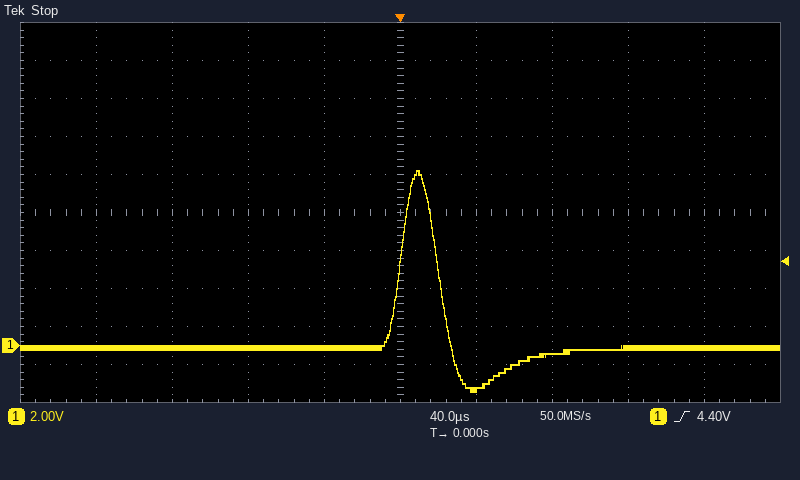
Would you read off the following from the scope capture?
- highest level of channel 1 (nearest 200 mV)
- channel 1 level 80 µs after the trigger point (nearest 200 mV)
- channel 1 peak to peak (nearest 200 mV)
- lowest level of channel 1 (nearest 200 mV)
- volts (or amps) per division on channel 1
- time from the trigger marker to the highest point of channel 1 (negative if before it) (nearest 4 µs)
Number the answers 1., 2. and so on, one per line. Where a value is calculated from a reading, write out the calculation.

1. 9.2 V
2. -400 mV
3. 9.2 V − (-2.4 V) = 11.6 V
4. -2.4 V
5. 2 V
6. +8 µs
